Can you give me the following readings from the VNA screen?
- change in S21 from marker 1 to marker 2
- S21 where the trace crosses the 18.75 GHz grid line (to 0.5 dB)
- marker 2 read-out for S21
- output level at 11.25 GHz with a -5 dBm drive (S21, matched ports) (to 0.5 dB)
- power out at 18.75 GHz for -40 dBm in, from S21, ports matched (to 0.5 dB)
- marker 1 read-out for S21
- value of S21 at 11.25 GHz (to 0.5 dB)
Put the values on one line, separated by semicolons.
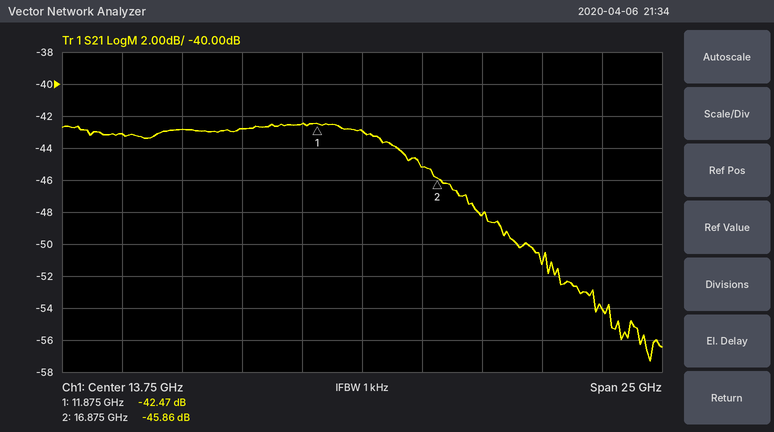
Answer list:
-3.39 dB; -48.0 dB; -45.86 dB; -47.5 dBm; -88.0 dBm; -42.47 dB; -42.5 dB
